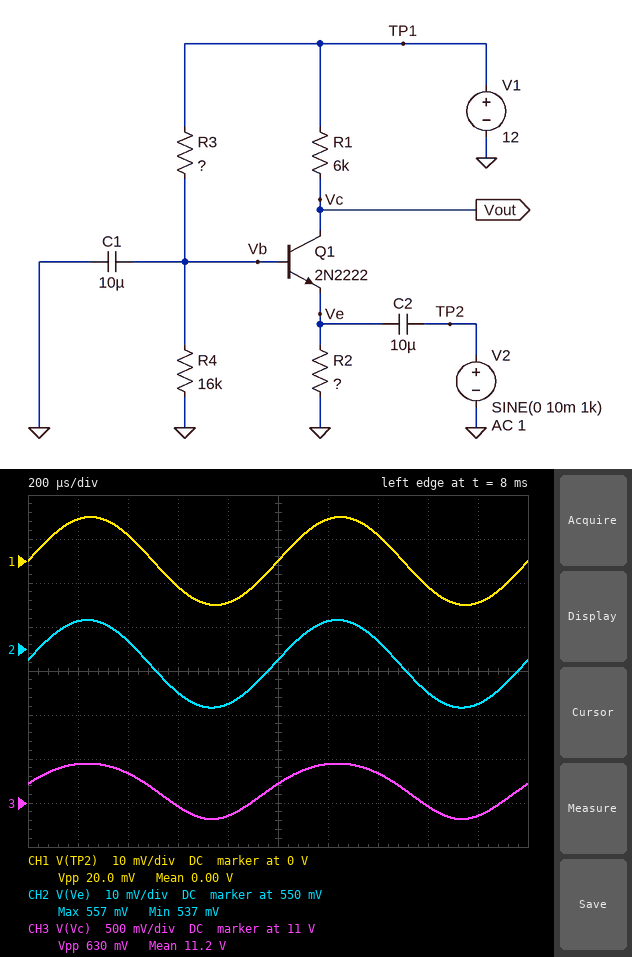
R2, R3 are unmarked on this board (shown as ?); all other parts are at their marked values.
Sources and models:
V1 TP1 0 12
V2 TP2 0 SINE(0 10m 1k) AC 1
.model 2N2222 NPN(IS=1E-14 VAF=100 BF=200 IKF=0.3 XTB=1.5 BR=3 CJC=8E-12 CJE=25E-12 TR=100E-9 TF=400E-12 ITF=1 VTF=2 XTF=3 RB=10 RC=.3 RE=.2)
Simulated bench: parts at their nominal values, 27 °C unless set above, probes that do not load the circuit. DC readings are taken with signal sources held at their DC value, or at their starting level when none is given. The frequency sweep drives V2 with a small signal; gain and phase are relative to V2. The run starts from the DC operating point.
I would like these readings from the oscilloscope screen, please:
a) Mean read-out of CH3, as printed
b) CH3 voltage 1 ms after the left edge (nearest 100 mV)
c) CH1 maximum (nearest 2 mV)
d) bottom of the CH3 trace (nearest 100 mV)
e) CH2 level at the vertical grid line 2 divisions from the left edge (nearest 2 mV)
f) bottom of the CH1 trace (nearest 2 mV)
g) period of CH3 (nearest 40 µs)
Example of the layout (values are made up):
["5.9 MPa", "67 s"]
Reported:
["11.2 V", "11.2 V", "10 mV", "10.8 V", "552 mV", "-10 mV", "1.00 ms"]
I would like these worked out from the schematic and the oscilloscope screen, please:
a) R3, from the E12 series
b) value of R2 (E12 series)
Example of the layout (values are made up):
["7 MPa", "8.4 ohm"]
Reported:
["150 kΩ", "3.9 kΩ"]
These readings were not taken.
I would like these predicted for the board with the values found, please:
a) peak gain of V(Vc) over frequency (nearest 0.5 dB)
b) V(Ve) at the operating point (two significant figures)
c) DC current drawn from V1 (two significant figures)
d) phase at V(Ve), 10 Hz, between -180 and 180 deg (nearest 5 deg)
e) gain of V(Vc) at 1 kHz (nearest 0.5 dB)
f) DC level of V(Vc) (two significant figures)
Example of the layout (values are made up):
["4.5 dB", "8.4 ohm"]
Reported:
["30.0 dB", "550 mV", "210 µA", "80 deg", "30.0 dB", "11 V"]
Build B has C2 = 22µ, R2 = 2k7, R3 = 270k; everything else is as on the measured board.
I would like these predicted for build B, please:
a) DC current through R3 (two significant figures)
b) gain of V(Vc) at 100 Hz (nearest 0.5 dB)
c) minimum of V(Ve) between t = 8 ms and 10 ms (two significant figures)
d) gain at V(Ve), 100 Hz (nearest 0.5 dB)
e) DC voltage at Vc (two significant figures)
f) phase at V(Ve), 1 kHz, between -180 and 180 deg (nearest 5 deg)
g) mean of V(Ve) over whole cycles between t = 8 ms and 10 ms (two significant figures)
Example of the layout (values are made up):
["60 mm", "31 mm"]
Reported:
["42 µA", "18.5 dB", "92 mV", "0 dB", "12 V", "0 deg", "100 mV"]
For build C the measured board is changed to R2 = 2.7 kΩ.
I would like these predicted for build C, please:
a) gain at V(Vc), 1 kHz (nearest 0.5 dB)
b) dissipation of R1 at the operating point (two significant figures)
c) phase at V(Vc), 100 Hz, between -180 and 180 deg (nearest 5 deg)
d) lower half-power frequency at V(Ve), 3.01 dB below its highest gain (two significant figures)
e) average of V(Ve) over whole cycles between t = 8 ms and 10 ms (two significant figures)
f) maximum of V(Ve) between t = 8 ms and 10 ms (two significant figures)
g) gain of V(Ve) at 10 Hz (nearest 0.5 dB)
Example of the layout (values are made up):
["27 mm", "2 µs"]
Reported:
["33.0 dB", "230 µW", "50 deg", "130 Hz", "530 mV", "540 mV", "-22.0 dB"]
